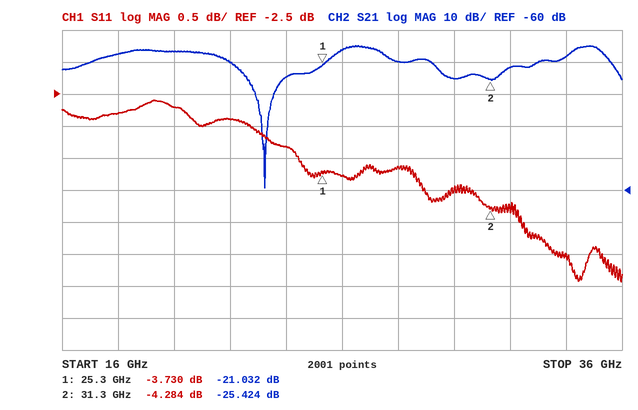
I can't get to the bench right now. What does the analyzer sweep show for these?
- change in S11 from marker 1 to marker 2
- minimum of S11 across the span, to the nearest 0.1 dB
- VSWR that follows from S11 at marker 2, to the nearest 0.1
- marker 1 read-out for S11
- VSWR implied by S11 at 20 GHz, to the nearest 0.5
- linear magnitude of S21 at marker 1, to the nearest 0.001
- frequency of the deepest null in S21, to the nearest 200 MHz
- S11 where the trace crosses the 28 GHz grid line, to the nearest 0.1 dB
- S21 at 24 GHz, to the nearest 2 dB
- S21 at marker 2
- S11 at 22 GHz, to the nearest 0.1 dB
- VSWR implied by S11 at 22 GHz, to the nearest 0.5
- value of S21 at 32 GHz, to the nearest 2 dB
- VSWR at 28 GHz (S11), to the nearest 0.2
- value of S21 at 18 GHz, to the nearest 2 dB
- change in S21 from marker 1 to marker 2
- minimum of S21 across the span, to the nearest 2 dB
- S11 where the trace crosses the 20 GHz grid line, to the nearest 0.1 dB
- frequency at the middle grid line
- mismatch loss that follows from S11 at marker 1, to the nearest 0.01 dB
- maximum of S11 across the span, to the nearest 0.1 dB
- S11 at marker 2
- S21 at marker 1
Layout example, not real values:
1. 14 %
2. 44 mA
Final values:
1. -0.554 dB
2. -5.4 dB
3. 4.1
4. -3.730 dB
5. 6.5
6. 0.089
7. 23.2 GHz
8. -3.6 dB
9. -24 dB
10. -25.424 dB
11. -2.9 dB
12. 6.0
13. -22 dB
14. 4.8
15. -18 dB
16. -4.392 dB
17. -60 dB
18. -2.7 dB
19. 26 GHz
20. 2.39 dB
21. -2.6 dB
22. -4.284 dB
23. -21.032 dB
